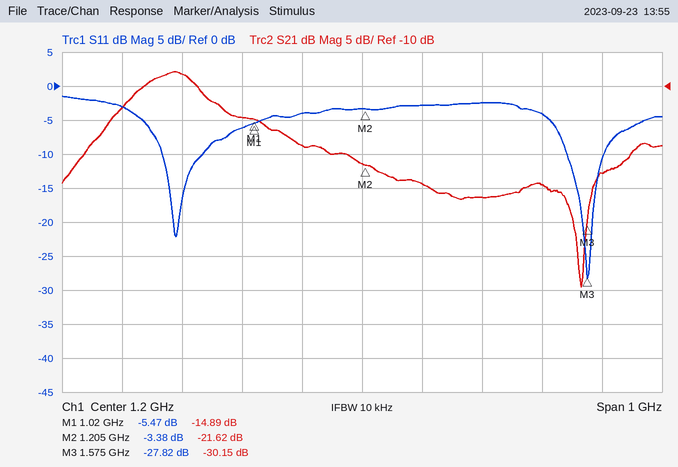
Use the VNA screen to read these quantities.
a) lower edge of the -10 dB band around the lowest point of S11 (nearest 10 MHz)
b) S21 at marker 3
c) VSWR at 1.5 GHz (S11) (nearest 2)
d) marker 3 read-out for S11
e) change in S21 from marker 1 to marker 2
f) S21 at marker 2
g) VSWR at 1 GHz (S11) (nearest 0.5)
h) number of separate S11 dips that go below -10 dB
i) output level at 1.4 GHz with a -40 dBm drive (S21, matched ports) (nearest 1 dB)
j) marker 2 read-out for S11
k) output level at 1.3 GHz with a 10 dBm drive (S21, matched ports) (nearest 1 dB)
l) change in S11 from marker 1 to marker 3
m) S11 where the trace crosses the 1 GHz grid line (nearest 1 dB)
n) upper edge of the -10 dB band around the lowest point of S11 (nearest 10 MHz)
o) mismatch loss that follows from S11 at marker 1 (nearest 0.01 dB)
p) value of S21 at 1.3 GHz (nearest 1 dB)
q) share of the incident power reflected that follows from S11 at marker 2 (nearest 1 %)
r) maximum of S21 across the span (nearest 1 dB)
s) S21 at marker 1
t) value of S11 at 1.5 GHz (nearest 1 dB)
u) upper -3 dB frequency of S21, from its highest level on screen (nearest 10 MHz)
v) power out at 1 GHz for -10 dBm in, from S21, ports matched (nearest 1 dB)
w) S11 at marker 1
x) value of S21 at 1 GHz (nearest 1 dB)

1.54 GHz
-30.15 dB
4
-27.82 dB
-6.73 dB
-21.62 dB
3.0
2
-66 dBm
-3.38 dB
-14 dBm
-22.35 dB
-6 dB
1.60 GHz
1.45 dB
-24 dB
46 %
-8 dB
-14.89 dB
-4 dB
930 MHz
-25 dBm
-5.47 dB
-15 dB
